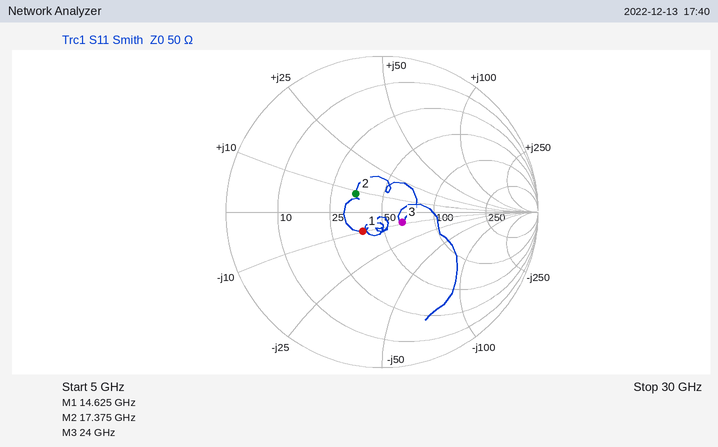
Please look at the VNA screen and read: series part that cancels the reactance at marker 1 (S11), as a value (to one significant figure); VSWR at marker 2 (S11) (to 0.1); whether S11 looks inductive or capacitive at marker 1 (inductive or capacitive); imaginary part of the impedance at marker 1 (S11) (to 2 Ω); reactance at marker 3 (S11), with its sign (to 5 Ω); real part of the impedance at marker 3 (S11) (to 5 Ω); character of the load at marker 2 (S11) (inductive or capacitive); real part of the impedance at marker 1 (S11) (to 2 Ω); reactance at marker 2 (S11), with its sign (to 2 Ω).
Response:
100 pH
1.5
capacitive
-10 Ω
-10 Ω
65 Ω
inductive
38 Ω
+8 Ω
